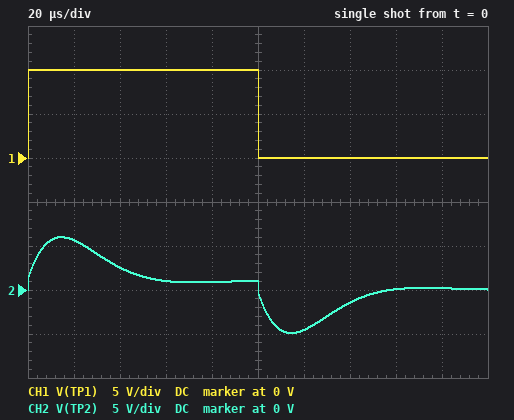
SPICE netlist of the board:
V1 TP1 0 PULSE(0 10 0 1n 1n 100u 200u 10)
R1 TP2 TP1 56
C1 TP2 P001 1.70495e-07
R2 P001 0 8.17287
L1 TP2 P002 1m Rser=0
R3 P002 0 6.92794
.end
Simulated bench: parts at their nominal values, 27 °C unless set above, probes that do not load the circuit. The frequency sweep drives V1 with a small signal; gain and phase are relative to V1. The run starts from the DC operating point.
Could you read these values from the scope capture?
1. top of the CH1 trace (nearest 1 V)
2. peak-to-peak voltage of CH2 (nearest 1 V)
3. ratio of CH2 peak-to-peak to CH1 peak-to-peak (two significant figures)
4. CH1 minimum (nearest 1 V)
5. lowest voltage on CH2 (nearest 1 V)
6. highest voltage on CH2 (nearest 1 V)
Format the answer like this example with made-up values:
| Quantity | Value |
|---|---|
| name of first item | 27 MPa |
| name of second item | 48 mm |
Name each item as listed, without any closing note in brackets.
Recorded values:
| Quantity | Value |
|---|---|
| top of the CH1 trace | 10 V |
| peak-to-peak voltage of CH2 | 11 V |
| ratio of CH2 peak-to-peak to CH1 peak-to-peak | 1.1 |
| CH1 minimum | 0 V |
| lowest voltage on CH2 | -5 V |
| highest voltage on CH2 | 6 V |
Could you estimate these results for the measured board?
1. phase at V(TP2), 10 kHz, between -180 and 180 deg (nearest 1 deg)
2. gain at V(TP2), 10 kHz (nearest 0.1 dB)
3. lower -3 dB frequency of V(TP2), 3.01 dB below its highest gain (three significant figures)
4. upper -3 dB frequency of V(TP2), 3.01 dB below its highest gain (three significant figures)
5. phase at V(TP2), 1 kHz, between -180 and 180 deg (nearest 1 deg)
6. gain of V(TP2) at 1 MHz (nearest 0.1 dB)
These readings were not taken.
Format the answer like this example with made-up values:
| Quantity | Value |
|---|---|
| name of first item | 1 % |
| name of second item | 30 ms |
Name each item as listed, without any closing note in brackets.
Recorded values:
| Quantity | Value |
|---|---|
| phase at V(TP2), 10 kHz, between -180 and 180 deg | 14 deg |
| gain at V(TP2), 10 kHz | -1.5 dB |
| lower -3 dB frequency of V(TP2), 3.01 dB below its highest gain | 6.26 kHz |
| upper -3 dB frequency of V(TP2), 3.01 dB below its highest gain | 23.4 kHz |
| phase at V(TP2), 1 kHz, between -180 and 180 deg | 36 deg |
| gain of V(TP2) at 1 MHz | -17.8 dB |
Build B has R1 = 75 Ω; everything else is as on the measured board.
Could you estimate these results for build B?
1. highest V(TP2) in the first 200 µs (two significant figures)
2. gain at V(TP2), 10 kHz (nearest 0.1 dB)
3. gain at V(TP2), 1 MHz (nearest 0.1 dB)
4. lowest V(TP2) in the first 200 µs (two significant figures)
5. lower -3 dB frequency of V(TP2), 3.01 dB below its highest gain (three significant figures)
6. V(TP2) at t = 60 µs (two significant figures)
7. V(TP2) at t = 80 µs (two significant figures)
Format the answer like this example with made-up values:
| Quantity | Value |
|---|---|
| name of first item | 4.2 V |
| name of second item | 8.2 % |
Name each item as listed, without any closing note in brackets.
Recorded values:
| Quantity | Value |
|---|---|
| highest V(TP2) in the first 200 µs | 5.2 V |
| gain at V(TP2), 10 kHz | -2.0 dB |
| gain at V(TP2), 1 MHz | -20.1 dB |
| lowest V(TP2) in the first 200 µs | -4.3 V |
| lower -3 dB frequency of V(TP2), 3.01 dB below its highest gain | 7.07 kHz |
| V(TP2) at t = 60 µs | 360 mV |
| V(TP2) at t = 80 µs | 530 mV |
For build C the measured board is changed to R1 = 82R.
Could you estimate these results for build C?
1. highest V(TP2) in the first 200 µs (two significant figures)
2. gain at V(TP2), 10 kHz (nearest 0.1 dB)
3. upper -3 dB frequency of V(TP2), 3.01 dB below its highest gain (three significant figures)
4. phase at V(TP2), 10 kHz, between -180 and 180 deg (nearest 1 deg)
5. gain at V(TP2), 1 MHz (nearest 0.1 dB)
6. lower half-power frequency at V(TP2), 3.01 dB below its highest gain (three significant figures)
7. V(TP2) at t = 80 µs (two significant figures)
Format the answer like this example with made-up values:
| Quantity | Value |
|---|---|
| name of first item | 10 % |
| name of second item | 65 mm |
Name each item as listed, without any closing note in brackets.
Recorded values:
| Quantity | Value |
|---|---|
| highest V(TP2) in the first 200 µs | 5.0 V |
| gain at V(TP2), 10 kHz | -2.2 dB |
| upper -3 dB frequency of V(TP2), 3.01 dB below its highest gain | 20.1 kHz |
| phase at V(TP2), 10 kHz, between -180 and 180 deg | 19 deg |
| gain at V(TP2), 1 MHz | -20.8 dB |
| lower half-power frequency at V(TP2), 3.01 dB below its highest gain | 7.31 kHz |
| V(TP2) at t = 80 µs | 440 mV |
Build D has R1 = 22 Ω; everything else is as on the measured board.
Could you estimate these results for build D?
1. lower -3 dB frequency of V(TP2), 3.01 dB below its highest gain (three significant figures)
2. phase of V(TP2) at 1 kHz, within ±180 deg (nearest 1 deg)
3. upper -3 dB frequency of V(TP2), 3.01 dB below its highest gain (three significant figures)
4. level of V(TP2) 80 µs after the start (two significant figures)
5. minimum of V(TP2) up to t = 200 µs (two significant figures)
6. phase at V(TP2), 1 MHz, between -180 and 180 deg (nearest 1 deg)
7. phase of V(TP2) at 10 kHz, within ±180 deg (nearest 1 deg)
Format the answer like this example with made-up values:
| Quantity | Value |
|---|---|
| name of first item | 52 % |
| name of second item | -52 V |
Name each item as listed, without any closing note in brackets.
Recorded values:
| Quantity | Value |
|---|---|
| lower -3 dB frequency of V(TP2), 3.01 dB below its highest gain | 3.66 kHz |
| phase of V(TP2) at 1 kHz, within ±180 deg | 30 deg |
| upper -3 dB frequency of V(TP2), 3.01 dB below its highest gain | 39.7 kHz |
| level of V(TP2) 80 µs after the start | 3.2 V |
| minimum of V(TP2) up to t = 200 µs | -5.4 V |
| phase at V(TP2), 1 MHz, between -180 and 180 deg | -5 deg |
| phase of V(TP2) at 10 kHz, within ±180 deg | 6 deg |
